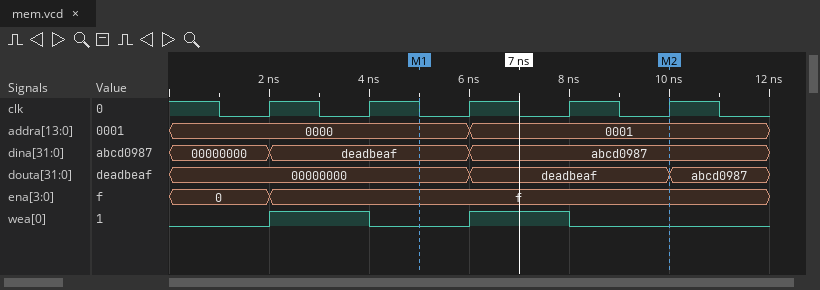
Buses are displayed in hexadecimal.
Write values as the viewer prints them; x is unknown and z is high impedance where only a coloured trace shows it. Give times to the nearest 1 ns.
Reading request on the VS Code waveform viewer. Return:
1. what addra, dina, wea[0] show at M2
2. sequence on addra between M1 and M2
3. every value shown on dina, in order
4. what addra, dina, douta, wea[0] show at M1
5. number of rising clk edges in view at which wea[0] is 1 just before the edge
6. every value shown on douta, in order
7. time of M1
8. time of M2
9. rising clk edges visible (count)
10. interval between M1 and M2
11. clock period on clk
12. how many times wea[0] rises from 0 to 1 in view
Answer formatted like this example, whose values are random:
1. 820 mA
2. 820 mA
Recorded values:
1. addra=0001, dina=abcd0987, wea[0]=0
2. 0000, 0001
3. 00000000, deadbeaf, abcd0987
4. addra=0000, dina=deadbeaf, douta=00000000, wea[0]=0
5. 2
6. 00000000, deadbeaf, abcd0987
7. 5 ns
8. 10 ns
9. 5
10. 5 ns
11. 2 ns
12. 2
